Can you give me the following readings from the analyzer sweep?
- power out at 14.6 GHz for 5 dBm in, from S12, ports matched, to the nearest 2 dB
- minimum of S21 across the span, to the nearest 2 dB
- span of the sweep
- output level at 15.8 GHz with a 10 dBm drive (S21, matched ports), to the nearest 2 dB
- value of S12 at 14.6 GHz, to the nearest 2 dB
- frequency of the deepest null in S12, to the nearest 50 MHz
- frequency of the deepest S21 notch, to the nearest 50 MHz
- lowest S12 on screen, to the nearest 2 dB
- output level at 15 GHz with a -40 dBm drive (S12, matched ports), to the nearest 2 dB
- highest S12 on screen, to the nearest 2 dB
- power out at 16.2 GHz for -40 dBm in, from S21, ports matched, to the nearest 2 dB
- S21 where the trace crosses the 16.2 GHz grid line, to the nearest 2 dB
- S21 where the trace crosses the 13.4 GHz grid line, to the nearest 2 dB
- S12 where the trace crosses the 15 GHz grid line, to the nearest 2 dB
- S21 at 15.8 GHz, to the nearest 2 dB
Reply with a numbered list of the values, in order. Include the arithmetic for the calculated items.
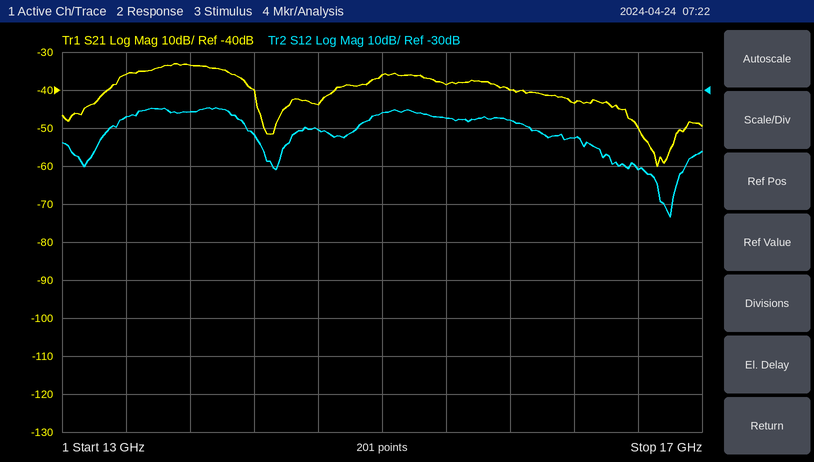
1. 5 dBm + (-40 dB) = -36 dBm
2. -60 dB
3. 4 GHz
4. 10 dBm + (-40 dB) = -30 dBm
5. -40 dB
6. 16.80 GHz
7. 16.70 GHz
8. -64 dB
9. -40 dBm + (-36 dB) = -76 dBm
10. -34 dB
11. -40 dBm + (-44 dB) = -84 dBm
12. -44 dB
13. -36 dB
14. -36 dB
15. -40 dB
